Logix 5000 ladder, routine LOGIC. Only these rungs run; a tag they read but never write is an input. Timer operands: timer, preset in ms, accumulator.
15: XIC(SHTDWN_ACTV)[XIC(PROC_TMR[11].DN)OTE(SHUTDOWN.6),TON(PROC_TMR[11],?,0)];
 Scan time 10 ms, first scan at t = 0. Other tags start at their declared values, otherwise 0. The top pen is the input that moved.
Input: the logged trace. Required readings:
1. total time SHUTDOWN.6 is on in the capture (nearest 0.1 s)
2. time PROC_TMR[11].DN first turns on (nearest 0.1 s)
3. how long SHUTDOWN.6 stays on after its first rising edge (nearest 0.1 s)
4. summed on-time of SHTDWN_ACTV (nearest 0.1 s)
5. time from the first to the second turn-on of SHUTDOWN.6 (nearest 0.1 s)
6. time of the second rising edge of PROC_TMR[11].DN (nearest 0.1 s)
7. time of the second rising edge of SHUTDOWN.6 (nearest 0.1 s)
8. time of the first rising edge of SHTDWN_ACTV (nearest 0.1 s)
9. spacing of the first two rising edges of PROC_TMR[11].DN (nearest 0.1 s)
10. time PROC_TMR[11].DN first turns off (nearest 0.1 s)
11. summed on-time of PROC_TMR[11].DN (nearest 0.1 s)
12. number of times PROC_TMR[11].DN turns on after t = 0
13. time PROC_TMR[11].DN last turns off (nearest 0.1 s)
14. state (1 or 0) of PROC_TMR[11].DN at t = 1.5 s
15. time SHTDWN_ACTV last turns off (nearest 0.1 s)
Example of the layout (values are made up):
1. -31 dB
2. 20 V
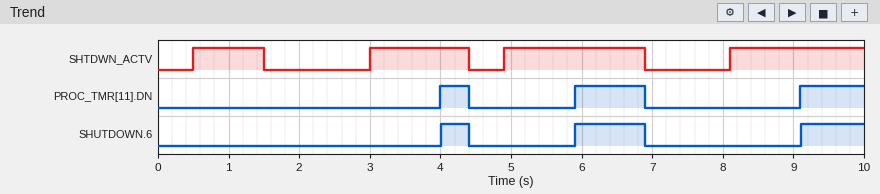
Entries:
1. 2.3 s
2. 4.0 s
3. 0.4 s
4. 6.3 s
5. 1.9 s
6. 5.9 s
7. 5.9 s
8. 0.5 s
9. 1.9 s
10. 4.4 s
11. 2.3 s
12. 3
13. 6.9 s
14. 0
15. 6.9 s
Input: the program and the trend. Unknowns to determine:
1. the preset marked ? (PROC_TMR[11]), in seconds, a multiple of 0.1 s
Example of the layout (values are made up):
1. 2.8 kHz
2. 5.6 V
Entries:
1. 1.0 s
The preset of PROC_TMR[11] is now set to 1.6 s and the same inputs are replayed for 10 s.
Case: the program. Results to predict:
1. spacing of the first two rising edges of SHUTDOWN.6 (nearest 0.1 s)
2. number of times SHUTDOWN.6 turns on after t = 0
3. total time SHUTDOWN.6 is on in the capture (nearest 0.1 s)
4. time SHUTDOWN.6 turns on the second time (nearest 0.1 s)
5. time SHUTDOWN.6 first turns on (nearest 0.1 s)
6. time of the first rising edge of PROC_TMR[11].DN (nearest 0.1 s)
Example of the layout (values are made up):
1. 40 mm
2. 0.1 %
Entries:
1. 3.2 s
2. 2
3. 0.7 s
4. 9.7 s
5. 6.5 s
6. 6.5 s
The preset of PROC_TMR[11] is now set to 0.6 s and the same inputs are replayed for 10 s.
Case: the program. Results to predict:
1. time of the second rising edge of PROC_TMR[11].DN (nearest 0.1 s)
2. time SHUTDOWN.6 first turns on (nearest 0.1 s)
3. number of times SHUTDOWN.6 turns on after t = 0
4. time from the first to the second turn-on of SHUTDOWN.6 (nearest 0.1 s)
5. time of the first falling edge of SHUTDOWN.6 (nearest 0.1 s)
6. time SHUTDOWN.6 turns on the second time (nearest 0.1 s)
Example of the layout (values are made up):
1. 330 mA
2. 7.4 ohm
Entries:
1. 3.6 s
2. 1.1 s
3. 4
4. 2.5 s
5. 1.5 s
6. 3.6 s
